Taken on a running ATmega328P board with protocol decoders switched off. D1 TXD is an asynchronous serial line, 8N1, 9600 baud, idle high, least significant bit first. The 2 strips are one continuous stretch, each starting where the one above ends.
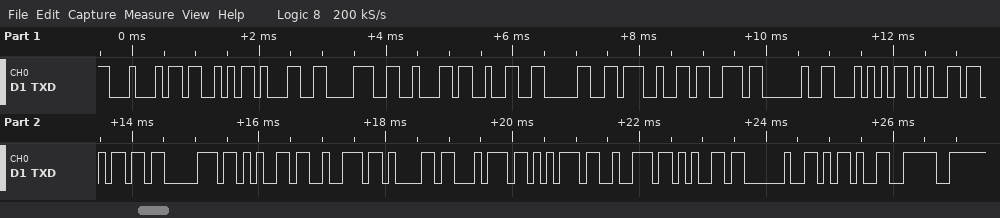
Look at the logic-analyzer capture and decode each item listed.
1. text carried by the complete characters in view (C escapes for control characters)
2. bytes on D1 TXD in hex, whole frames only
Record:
"DS18b20's Temperature ->"
44 53 31 38 62 32 30 27 73 20 54 65 6D 70 65 72 61 74 75 72 65 20 2D 3E
